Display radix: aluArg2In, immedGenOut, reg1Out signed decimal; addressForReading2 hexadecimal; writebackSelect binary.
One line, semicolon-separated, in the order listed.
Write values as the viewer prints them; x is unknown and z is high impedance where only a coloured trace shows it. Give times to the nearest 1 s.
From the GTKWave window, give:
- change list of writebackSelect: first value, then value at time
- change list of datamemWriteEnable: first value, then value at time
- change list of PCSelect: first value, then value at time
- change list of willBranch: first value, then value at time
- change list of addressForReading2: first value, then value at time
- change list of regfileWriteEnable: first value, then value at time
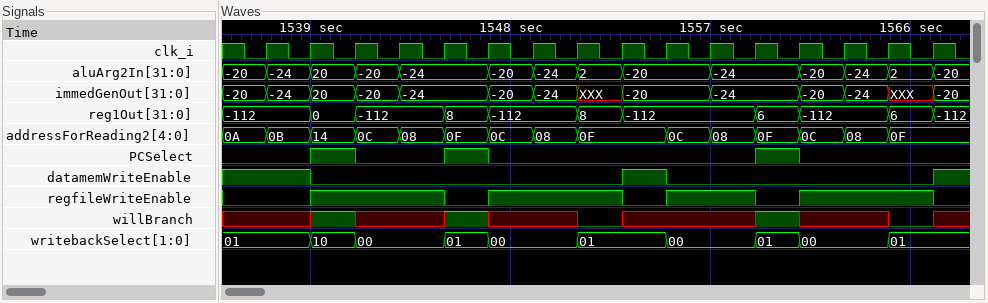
01, 10 at 1539 s, 00 at 1541 s, 01 at 1545 s, 00 at 1547 s, 01 at 1551 s, 00 at 1555 s, 01 at 1559 s, 00 at 1561 s, 01 at 1565 s; 1, 0 at 1539 s, 1 at 1553 s, 0 at 1555 s, 1 at 1567 s; 0, 1 at 1539 s, 0 at 1541 s, 1 at 1545 s, 0 at 1547 s, 1 at 1559 s, 0 at 1561 s; x, 1 at 1539 s, x at 1541 s, 1 at 1545 s, x at 1547 s, 0 at 1551 s, x at 1553 s, 1 at 1559 s, x at 1561 s, 0 at 1565 s, x at 1567 s; 0A, 0B at 1537 s, 14 at 1539 s, 0C at 1541 s, 08 at 1543 s, 0F at 1545 s, 0C at 1547 s, 08 at 1549 s, 0F at 1551 s, 0C at 1555 s, 08 at 1557 s, 0F at 1559 s, 0C at 1561 s, 08 at 1563 s, 0F at 1565 s; 0, 1 at 1539 s, 0 at 1545 s, 1 at 1547 s, 0 at 1553 s, 1 at 1555 s, 0 at 1559 s, 1 at 1561 s, 0 at 1567 s
